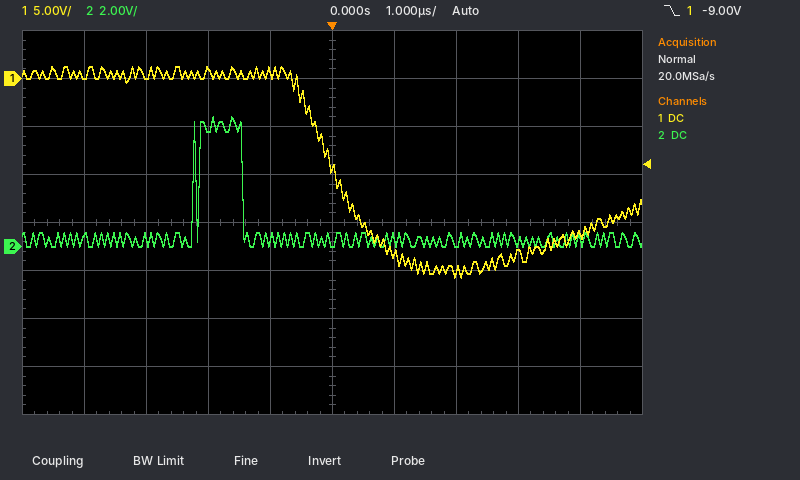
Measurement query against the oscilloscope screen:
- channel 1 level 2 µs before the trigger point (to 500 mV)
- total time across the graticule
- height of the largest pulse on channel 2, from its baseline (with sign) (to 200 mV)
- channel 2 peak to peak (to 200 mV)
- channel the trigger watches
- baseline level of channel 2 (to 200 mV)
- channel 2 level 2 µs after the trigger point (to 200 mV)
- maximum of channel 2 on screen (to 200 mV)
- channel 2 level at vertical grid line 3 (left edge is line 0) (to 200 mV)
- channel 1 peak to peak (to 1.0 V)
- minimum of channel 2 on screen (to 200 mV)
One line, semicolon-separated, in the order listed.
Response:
1.0 V; 10 µs; +5.2 V; 5.4 V; channel 1; 200 mV; 200 mV; 5.4 V; 5.0 V; 22.0 V; 0.0 V
